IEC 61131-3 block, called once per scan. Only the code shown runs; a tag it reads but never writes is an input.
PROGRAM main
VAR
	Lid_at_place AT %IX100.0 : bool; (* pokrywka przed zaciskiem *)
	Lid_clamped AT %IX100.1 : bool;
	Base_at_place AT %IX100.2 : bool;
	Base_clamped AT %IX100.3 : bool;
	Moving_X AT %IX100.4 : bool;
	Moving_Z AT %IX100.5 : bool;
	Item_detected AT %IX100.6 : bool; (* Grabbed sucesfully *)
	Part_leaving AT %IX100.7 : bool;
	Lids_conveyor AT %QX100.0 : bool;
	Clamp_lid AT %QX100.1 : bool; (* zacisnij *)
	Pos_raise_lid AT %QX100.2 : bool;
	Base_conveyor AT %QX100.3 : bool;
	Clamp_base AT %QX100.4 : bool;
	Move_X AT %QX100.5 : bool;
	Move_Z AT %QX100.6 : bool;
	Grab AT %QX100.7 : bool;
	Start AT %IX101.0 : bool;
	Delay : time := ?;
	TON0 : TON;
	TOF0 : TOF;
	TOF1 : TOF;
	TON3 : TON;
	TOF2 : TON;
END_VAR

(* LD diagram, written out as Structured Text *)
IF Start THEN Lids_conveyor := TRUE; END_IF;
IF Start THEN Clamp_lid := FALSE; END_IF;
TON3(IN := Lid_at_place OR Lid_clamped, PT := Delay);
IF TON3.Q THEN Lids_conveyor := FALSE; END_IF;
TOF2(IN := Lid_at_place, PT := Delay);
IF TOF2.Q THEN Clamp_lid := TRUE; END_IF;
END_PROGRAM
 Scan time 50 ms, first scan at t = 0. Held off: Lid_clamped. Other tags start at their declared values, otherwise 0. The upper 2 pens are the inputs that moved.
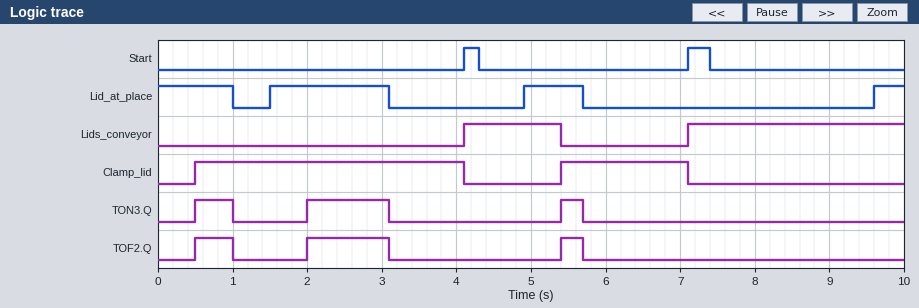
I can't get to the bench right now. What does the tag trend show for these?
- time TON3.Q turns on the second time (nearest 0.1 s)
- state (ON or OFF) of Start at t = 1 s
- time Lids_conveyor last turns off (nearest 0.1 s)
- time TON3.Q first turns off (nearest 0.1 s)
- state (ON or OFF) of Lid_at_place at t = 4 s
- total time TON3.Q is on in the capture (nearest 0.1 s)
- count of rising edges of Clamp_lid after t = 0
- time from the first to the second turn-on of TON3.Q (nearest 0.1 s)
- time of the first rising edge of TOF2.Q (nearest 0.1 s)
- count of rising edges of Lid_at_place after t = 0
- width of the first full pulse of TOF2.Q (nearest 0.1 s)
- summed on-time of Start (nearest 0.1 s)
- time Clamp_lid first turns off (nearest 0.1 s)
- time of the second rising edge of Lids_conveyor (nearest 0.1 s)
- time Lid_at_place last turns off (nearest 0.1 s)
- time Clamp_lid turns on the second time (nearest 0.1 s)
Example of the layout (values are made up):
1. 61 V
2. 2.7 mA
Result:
1. 2.0 s
2. OFF
3. 5.4 s
4. 1.0 s
5. OFF
6. 1.9 s
7. 2
8. 1.5 s
9. 0.5 s
10. 3
11. 0.5 s
12. 0.5 s
13. 4.1 s
14. 7.1 s
15. 5.7 s
16. 5.4 s
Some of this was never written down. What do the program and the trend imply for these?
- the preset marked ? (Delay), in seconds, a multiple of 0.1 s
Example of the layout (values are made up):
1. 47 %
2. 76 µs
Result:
1. 0.5 s
